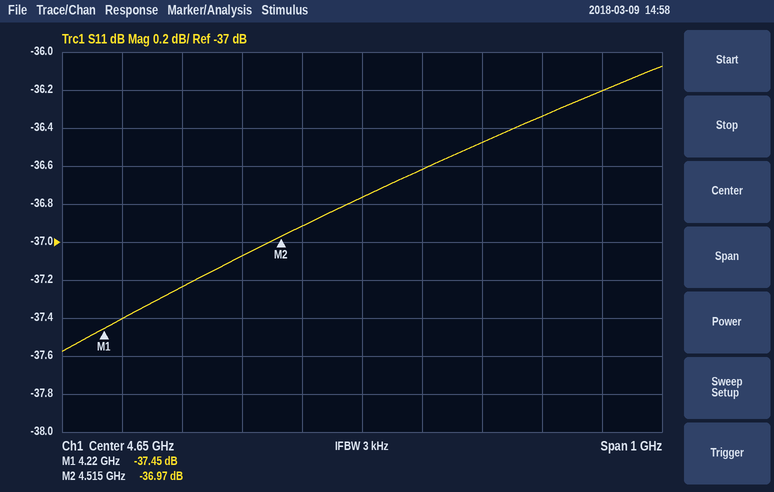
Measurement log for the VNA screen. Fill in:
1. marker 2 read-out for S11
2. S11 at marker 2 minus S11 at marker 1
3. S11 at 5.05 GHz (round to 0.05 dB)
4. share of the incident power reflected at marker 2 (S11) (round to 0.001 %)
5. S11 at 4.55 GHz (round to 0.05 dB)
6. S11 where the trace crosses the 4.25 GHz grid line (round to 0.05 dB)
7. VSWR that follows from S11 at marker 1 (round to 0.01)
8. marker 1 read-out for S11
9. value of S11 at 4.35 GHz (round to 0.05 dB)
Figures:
-36.97 dB
0.48 dB
-36.20 dB
0.020 %
-36.90 dB
-37.40 dB
1.03
-37.45 dB
-37.25 dB
